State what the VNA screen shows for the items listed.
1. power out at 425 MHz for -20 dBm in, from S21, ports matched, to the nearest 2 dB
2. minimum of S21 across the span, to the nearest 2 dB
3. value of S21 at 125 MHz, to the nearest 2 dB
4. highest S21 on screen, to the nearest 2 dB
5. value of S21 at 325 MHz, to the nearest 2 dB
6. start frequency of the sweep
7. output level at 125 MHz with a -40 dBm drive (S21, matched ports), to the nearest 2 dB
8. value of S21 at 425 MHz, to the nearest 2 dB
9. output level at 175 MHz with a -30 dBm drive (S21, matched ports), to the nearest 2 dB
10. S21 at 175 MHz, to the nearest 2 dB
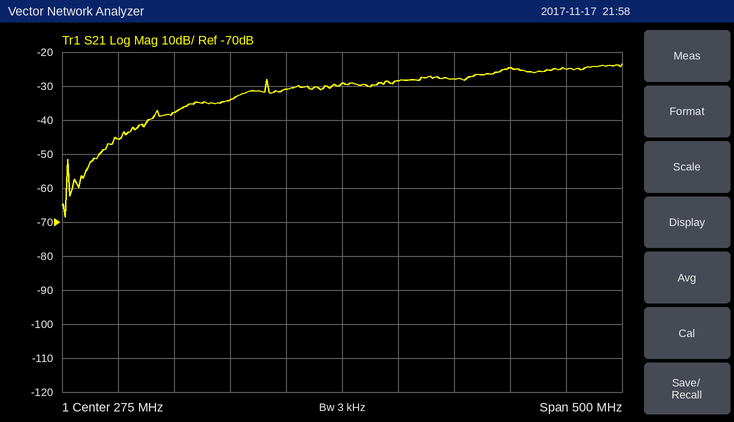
-44 dBm
-68 dB
-38 dB
-24 dB
-28 dB
25 MHz
-78 dBm
-24 dB
-64 dBm
-34 dB
